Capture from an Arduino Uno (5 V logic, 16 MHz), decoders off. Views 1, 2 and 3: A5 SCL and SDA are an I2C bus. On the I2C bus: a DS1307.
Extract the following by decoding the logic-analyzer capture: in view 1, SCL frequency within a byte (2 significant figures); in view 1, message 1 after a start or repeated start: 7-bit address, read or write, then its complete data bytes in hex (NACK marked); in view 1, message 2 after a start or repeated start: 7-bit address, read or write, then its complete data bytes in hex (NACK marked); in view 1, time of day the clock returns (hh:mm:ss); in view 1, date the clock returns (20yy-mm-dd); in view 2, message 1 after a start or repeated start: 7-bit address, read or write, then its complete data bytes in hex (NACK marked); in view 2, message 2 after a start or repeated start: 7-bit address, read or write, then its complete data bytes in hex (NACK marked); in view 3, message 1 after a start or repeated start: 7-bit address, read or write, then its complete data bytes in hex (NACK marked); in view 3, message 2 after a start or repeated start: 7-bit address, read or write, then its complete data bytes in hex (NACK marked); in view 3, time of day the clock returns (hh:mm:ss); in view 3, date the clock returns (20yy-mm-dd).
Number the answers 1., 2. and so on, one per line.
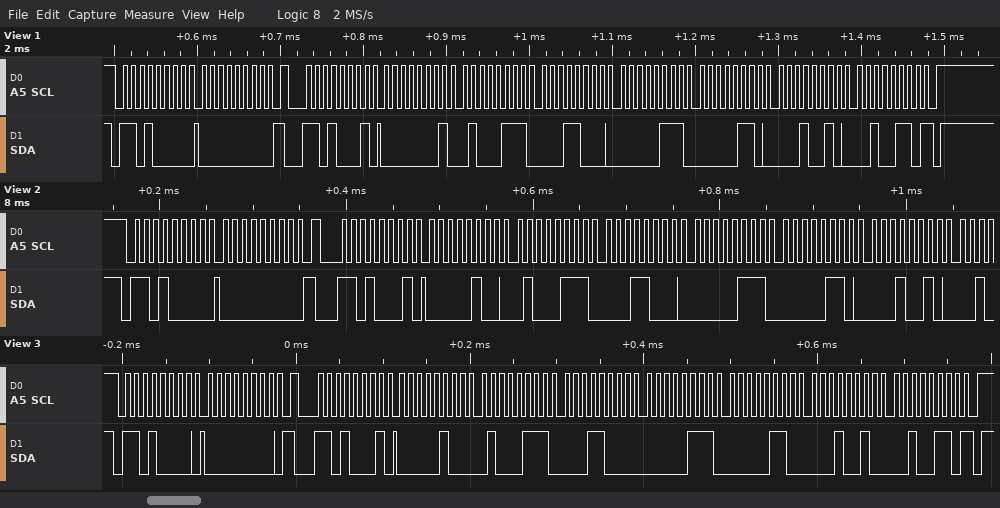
1. 100 kHz
2. 0x68 write: 00
3. 0x68 read: 01 47 18 07 06 12 26 NACK
4. 18:47:01
5. 2026-12-06
6. 0x68 write: 00
7. 0x68 read: 04 47 18 07 06 12
8. 0x68 write: 00
9. 0x68 read: 04 47 18 07 06 12 26 NACK
10. 18:47:04
11. 2026-12-06
